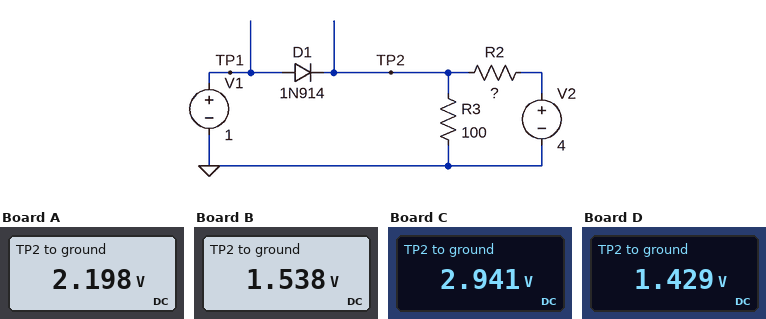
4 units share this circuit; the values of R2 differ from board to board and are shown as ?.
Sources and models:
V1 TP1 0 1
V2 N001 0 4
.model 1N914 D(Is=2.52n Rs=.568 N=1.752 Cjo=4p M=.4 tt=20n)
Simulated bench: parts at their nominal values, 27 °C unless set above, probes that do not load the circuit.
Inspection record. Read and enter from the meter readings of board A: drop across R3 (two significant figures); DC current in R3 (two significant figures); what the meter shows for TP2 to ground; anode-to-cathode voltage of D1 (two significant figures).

2.2 V
22 mA
2.198 V
-1.2 V
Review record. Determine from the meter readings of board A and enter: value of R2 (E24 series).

82 Ω
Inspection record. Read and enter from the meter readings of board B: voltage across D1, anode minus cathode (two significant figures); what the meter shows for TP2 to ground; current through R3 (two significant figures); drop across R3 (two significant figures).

-540 mV
1.538 V
15 mA
1.5 V
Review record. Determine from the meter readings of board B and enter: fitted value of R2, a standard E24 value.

160 Ω
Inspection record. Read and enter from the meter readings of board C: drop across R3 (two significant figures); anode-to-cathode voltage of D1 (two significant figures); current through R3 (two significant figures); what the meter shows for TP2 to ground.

2.9 V
-1.9 V
29 mA
2.941 V
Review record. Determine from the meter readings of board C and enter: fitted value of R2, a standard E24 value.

36 Ω
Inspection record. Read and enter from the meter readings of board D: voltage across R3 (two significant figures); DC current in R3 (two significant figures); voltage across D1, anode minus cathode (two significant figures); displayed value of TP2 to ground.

1.4 V
14 mA
-430 mV
1.429 V
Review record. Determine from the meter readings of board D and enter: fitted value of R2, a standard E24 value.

180 Ω
